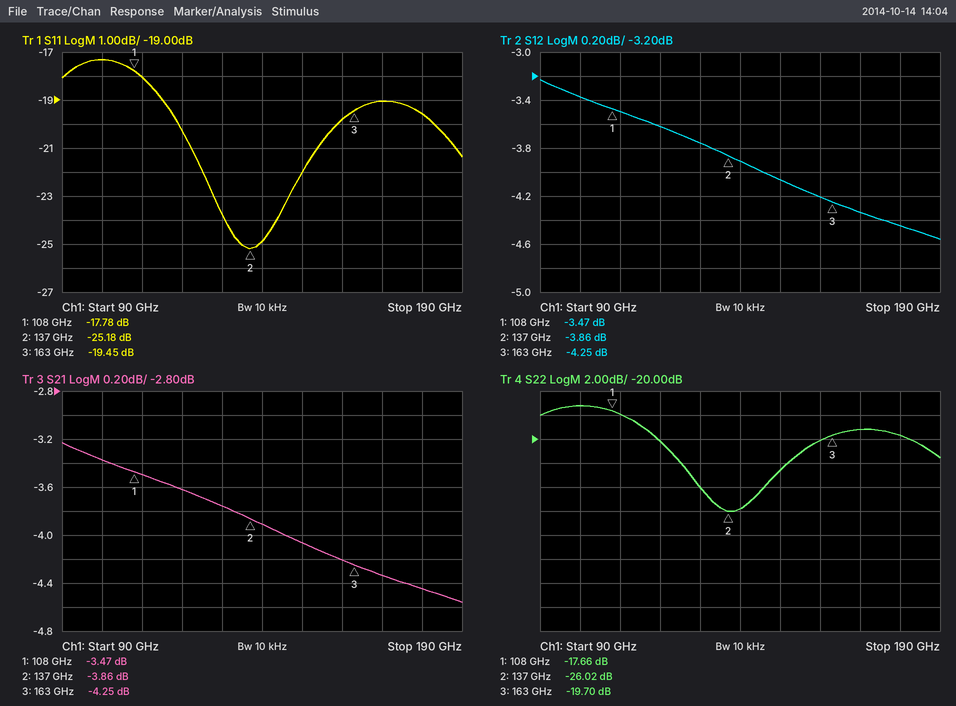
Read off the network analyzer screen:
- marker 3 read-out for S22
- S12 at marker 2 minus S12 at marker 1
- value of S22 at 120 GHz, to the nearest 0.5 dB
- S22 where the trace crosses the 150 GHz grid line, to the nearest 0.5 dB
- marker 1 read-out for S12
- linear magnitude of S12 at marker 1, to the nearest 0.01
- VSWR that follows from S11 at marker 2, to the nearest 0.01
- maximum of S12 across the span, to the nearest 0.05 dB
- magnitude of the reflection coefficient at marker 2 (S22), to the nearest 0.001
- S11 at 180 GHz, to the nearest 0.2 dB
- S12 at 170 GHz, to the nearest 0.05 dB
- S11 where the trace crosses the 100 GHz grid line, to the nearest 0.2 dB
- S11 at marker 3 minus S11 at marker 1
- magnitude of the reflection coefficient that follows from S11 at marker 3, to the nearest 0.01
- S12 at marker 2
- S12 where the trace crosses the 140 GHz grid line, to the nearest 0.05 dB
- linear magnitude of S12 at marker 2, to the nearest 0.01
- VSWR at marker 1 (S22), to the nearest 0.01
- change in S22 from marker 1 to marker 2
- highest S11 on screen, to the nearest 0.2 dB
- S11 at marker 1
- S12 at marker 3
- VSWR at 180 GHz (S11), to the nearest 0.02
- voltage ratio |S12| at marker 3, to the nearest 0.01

-19.70 dB
-0.39 dB
-20.0 dB
-22.5 dB
-3.47 dB
0.67
1.12
-3.25 dB
0.050
-19.6 dB
-4.35 dB
-17.4 dB
-1.67 dB
0.11
-3.86 dB
-3.90 dB
0.64
1.30
-8.36 dB
-17.4 dB
-17.78 dB
-4.25 dB
1.24
0.61
